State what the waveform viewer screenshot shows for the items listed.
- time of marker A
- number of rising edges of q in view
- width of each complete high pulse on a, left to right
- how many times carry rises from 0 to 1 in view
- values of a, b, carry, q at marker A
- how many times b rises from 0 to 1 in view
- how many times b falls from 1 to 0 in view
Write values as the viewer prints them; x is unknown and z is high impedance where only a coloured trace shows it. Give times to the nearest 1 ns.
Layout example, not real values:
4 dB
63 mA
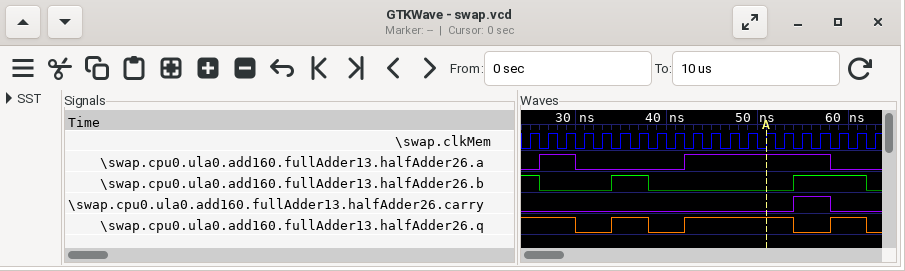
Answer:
51 ns
3
4 ns, 16 ns
1
a=1, b=0, carry=0, q=1
2
3
